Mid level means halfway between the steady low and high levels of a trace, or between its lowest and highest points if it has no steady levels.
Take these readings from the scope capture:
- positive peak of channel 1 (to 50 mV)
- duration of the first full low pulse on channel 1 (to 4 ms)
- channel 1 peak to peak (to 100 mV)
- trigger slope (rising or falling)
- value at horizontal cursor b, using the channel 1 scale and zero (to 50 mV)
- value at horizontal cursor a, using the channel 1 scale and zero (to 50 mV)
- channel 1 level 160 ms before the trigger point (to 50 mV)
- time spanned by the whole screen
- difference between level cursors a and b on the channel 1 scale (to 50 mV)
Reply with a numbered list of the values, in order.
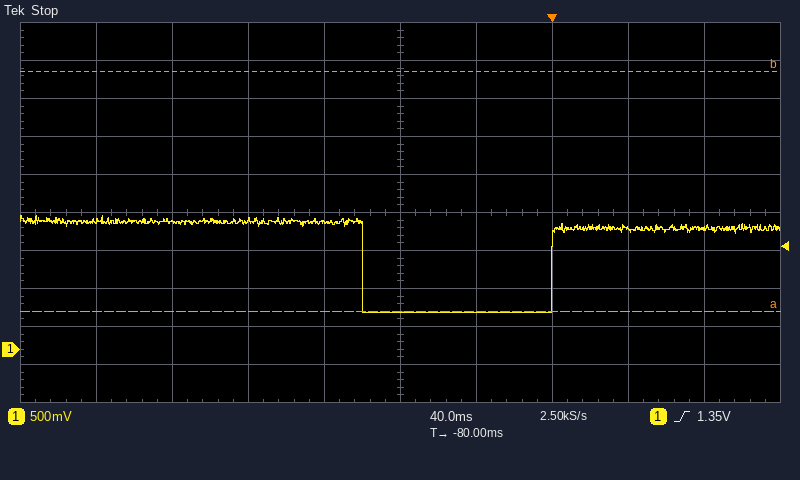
1. 1.75 V
2. 100 ms
3. 1.30 V
4. rising
5. 3.65 V
6. 500 mV
7. 1.70 V
8. 400 ms
9. 3.15 V
